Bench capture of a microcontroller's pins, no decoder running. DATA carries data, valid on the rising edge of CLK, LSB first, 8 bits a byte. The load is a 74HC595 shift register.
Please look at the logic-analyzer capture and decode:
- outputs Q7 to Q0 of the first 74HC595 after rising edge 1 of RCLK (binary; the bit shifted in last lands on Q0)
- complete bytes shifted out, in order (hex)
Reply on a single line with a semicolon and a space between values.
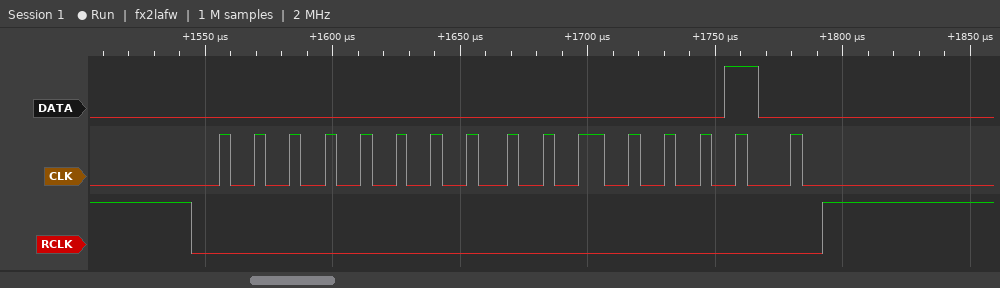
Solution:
00000010; 00 40
